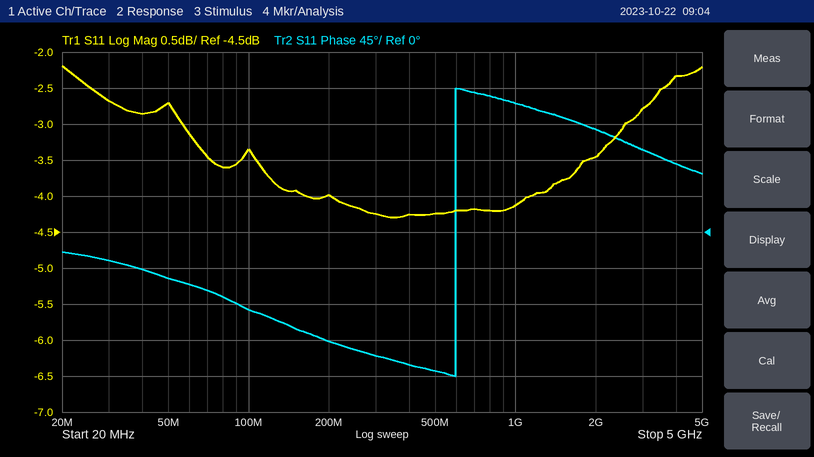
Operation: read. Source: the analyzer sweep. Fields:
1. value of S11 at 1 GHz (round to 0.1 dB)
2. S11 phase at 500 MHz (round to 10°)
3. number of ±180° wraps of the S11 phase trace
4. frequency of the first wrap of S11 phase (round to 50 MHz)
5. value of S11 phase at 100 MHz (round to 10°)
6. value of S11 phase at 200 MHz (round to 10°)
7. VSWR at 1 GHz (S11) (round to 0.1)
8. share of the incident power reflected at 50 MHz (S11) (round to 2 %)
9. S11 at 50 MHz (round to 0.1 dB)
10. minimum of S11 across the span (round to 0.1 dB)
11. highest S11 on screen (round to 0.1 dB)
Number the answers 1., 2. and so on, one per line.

1. -4.1 dB
2. -170°
3. 1
4. 600 MHz
5. -100°
6. -140°
7. 4.3
8. 54 %
9. -2.7 dB
10. -4.3 dB
11. -2.2 dB
